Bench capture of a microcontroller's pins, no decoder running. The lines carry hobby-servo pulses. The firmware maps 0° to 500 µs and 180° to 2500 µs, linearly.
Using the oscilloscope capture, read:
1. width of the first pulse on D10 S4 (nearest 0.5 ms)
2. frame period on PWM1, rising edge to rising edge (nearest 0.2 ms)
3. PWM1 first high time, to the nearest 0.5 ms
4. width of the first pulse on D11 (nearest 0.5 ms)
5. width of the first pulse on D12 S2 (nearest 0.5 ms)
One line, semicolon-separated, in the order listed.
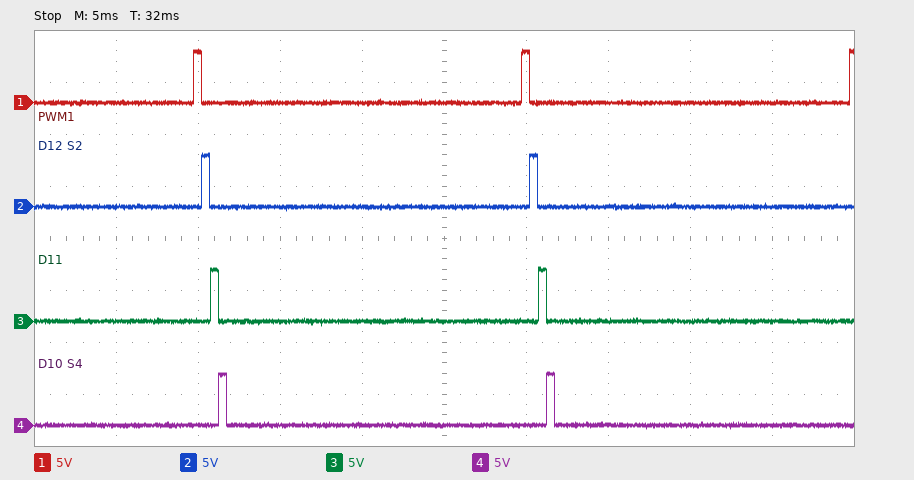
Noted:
0.5 ms; 20.0 ms; 0.5 ms; 0.5 ms; 0.5 ms
